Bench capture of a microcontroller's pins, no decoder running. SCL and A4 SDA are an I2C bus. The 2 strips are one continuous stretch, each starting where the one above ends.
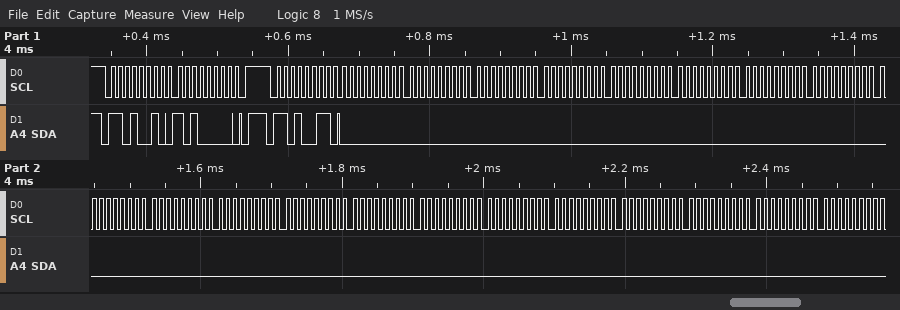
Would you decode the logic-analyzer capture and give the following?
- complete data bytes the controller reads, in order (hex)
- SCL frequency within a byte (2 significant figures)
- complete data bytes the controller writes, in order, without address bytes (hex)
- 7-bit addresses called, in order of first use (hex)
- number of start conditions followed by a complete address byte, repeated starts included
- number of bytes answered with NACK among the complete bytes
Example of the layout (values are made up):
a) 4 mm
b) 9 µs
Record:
a) 00 00 00 00 00 00 00 00 00 00 00 00 00 00 00 00 00 00 00 00
b) 100 kHz
c) A0
d) 0x69
e) 2
f) 0
